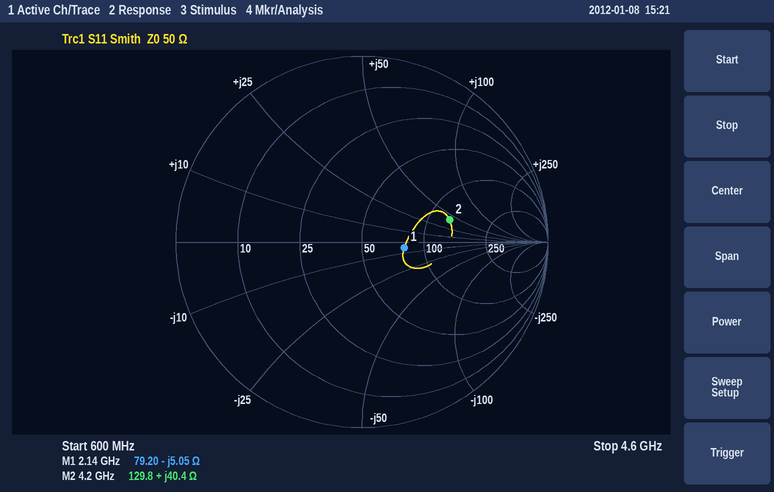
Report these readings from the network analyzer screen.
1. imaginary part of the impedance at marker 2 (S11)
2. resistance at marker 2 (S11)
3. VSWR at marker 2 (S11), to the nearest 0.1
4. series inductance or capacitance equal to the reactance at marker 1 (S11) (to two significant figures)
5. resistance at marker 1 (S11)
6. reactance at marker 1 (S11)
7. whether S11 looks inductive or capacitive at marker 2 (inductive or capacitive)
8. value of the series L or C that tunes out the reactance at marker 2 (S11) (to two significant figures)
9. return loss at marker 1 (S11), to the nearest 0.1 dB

+40.4 Ω
129.8 Ω
2.9
15 pF
79.20 Ω
-5.05 Ω
inductive
940 fF
12.8 dB
